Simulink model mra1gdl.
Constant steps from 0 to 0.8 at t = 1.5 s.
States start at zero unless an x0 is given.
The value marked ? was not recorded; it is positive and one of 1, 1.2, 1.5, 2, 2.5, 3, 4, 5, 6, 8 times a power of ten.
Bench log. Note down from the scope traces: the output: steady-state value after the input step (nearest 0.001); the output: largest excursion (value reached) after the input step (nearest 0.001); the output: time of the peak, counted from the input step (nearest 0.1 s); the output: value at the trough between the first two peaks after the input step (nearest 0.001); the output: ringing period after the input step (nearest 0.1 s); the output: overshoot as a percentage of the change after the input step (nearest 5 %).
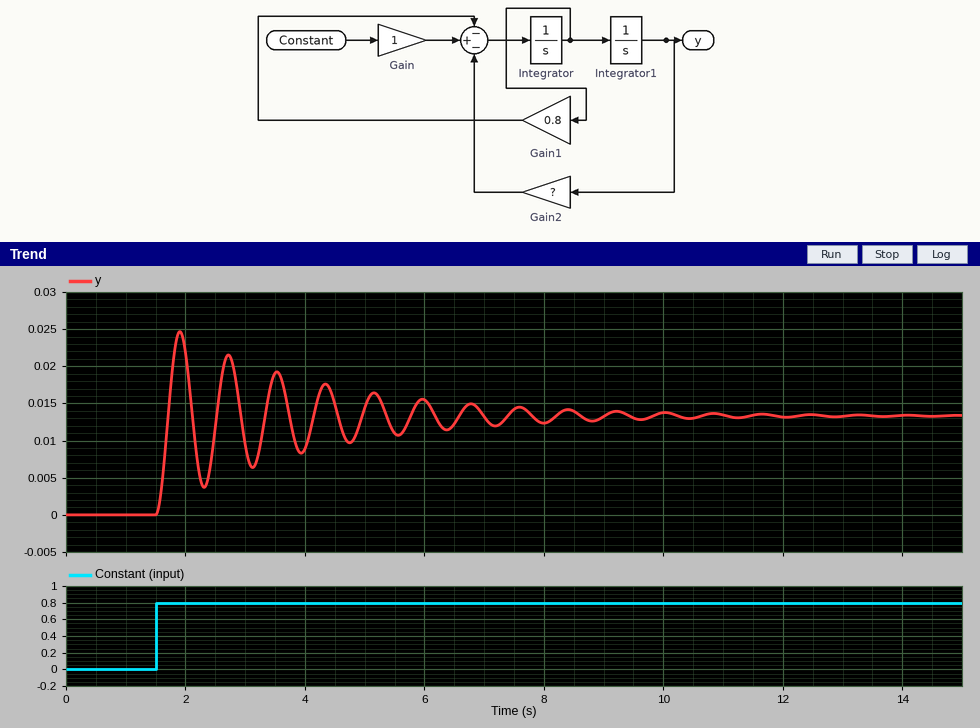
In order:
0.013
0.025
0.4 s
0.004
0.8 s
85 %
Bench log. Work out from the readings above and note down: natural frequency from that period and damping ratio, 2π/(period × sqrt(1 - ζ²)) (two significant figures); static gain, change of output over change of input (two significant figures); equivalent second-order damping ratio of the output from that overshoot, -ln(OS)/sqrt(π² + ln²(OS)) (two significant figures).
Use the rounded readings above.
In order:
7.9 rad/s
0.016
0.052
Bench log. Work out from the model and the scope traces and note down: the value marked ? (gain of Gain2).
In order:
60
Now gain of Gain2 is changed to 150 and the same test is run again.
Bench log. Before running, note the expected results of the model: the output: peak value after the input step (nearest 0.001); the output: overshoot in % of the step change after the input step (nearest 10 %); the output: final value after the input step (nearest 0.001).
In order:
0.010
90 %
0.005
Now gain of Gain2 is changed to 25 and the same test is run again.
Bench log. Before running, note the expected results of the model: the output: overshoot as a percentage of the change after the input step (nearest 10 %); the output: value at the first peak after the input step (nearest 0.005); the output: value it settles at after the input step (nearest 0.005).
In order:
80 %
0.055
0.030
